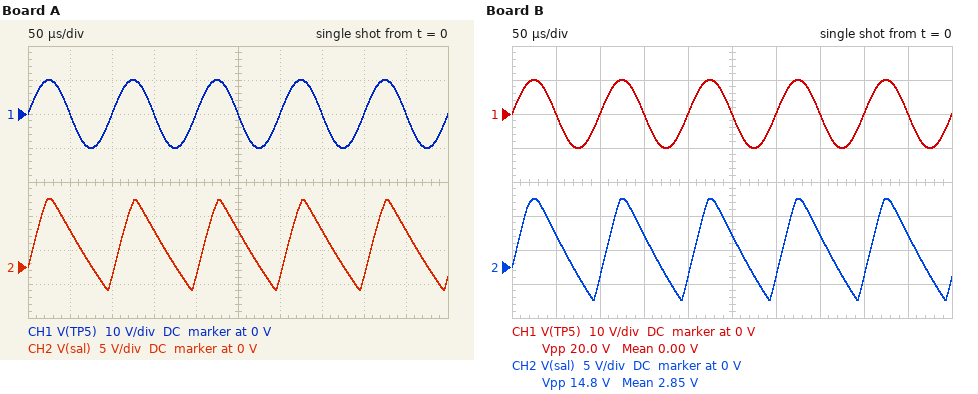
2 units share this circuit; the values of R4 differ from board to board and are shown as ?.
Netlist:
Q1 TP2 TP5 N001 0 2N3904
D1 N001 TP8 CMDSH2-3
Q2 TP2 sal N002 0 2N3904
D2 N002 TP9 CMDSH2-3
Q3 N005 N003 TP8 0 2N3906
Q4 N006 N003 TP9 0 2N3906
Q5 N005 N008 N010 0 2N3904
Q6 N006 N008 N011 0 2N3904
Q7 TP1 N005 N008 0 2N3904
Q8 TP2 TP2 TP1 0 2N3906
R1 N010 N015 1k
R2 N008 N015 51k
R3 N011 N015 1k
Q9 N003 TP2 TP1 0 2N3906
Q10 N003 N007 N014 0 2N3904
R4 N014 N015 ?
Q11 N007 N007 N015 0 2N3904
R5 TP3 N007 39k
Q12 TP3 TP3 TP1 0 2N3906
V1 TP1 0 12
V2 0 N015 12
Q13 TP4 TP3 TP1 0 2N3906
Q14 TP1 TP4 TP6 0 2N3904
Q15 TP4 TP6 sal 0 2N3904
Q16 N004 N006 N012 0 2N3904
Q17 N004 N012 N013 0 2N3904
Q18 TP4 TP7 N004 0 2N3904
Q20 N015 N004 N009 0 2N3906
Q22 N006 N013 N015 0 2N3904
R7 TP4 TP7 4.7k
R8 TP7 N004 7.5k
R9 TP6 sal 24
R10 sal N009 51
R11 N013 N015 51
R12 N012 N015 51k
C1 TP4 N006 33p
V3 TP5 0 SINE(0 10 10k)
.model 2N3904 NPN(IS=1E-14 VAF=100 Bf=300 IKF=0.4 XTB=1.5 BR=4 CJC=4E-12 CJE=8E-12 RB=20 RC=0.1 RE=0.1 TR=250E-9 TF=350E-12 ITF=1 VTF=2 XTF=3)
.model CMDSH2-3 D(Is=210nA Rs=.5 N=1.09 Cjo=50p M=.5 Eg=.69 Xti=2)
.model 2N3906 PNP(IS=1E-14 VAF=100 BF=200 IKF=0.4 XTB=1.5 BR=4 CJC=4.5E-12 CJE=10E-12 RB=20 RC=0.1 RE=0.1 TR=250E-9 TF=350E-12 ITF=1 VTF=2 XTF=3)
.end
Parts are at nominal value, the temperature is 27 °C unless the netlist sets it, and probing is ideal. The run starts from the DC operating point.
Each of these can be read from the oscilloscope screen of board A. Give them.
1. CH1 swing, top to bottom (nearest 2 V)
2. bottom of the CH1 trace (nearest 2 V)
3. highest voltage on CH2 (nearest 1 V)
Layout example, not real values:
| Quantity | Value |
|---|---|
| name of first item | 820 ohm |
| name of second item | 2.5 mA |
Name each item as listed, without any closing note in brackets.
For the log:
| Quantity | Value |
|---|---|
| CH1 swing, top to bottom | 20 V |
| bottom of the CH1 trace | -10 V |
| highest voltage on CH2 | 10 V |
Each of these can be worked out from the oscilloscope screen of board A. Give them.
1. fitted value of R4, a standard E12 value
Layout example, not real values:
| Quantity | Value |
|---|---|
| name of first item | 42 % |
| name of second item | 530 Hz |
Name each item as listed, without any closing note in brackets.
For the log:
| Quantity | Value |
|---|---|
| fitted value of R4, a standard E12 value | 10 kΩ |
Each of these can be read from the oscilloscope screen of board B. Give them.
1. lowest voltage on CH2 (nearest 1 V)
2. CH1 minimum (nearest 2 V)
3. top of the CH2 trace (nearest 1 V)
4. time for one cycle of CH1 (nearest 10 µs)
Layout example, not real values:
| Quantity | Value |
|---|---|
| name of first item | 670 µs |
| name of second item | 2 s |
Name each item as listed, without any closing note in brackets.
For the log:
| Quantity | Value |
|---|---|
| lowest voltage on CH2 | -5 V |
| CH1 minimum | -10 V |
| top of the CH2 trace | 10 V |
| time for one cycle of CH1 | 100 µs |
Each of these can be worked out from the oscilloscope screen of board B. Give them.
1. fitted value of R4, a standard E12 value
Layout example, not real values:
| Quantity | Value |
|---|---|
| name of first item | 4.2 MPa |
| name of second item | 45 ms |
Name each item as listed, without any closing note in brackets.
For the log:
| Quantity | Value |
|---|---|
| fitted value of R4, a standard E12 value | 8.2 kΩ |
